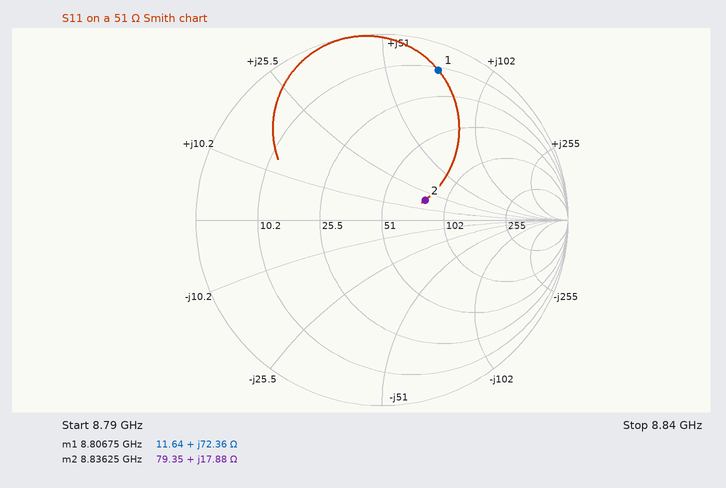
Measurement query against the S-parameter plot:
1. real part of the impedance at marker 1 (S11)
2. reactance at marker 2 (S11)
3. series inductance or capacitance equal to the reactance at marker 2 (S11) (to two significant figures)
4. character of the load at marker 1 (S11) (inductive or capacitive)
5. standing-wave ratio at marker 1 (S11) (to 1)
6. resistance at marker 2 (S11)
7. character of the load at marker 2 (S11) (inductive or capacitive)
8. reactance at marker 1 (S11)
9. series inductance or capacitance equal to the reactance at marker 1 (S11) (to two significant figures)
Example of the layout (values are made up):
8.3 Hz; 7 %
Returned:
11.64 Ω; +17.88 Ω; 320 pH; inductive; 13; 79.35 Ω; inductive; +72.36 Ω; 1.3 nH
